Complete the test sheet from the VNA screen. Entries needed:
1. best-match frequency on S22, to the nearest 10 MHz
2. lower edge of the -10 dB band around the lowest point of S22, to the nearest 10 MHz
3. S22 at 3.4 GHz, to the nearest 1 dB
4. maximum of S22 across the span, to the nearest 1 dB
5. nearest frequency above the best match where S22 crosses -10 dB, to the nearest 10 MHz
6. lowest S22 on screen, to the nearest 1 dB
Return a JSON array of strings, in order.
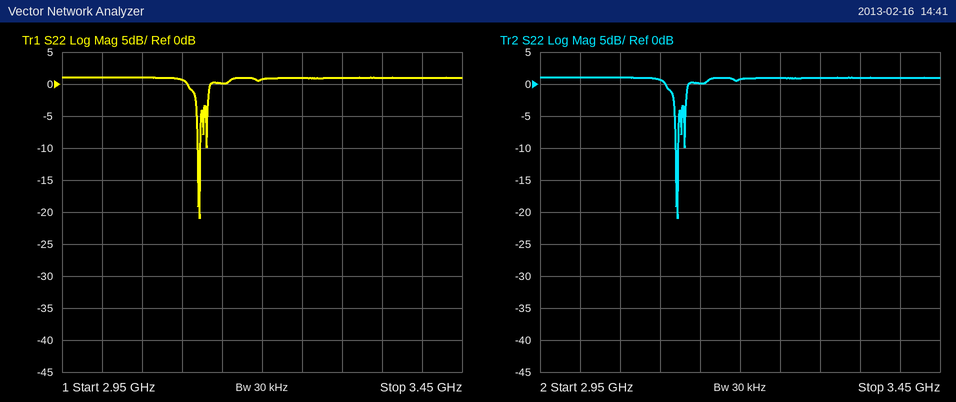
["3.12 GHz", "3.12 GHz", "1 dB", "1 dB", "3.12 GHz", "-21 dB"]
